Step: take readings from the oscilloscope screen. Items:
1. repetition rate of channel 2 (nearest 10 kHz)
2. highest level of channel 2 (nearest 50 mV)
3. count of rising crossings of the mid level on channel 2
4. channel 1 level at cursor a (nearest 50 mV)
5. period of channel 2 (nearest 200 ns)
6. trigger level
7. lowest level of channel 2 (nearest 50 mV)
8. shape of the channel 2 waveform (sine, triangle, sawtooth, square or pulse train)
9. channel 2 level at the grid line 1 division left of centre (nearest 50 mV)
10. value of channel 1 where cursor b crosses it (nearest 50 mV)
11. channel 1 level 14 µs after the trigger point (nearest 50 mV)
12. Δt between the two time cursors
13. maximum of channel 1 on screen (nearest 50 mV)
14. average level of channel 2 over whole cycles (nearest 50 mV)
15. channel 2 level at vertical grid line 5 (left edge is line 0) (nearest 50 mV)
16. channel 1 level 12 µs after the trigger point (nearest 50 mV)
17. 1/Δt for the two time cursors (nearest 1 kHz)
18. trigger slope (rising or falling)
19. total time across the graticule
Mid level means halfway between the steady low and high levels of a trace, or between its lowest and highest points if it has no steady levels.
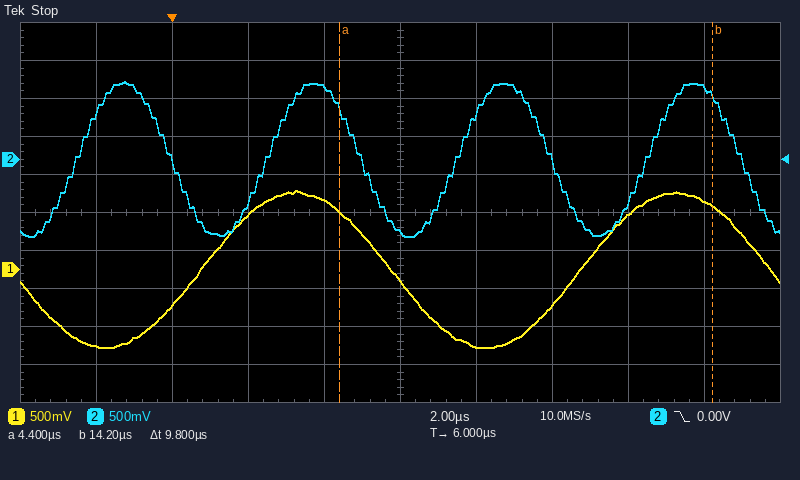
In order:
200 kHz
1.00 V
4
750 mV
5.0 µs
0.00 V
-1.00 V
sine
950 mV
850 mV
900 mV
9.8 µs
1.05 V
0 mV
-950 mV
700 mV
102 kHz
falling
20 µs
